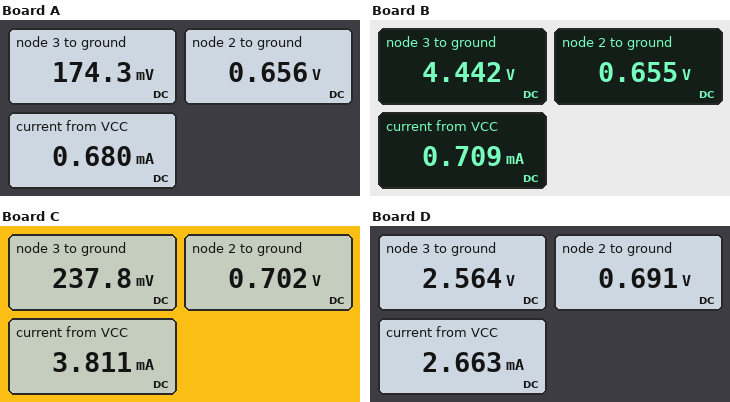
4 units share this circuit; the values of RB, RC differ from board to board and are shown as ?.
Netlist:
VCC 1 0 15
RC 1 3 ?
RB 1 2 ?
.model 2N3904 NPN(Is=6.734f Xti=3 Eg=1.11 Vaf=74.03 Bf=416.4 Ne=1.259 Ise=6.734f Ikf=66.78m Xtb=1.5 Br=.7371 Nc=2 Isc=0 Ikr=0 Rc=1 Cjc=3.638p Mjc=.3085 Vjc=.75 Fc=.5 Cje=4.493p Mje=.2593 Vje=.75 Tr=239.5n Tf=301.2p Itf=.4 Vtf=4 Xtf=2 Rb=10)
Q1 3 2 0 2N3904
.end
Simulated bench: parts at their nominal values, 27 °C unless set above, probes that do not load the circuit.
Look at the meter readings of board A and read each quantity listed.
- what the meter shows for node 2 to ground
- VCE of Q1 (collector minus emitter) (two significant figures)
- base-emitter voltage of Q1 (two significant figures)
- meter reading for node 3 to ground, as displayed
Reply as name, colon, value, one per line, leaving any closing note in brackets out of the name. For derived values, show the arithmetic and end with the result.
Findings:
what the meter shows for node 2 to ground: 0.656 V
VCE of Q1 (collector minus emitter): 174.3 mV = 170 mV
base-emitter voltage of Q1: 656 mV = 660 mV
meter reading for node 3 to ground, as displayed: 174.3 mV
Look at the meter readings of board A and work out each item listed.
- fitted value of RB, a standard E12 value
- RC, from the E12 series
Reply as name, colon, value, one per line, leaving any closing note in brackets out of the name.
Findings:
fitted value of RB, a standard E12 value: 2.2 MΩ
RC, from the E12 series: 22 kΩ
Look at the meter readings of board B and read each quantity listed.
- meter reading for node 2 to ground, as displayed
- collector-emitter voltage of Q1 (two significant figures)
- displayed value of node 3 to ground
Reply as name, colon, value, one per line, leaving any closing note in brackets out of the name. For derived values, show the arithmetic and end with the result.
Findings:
meter reading for node 2 to ground, as displayed: 0.655 V
collector-emitter voltage of Q1: 4.442 V = 4.4 V
displayed value of node 3 to ground: 4.442 V
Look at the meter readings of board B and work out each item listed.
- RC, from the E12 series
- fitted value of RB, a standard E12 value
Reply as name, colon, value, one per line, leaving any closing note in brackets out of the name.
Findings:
RC, from the E12 series: 15 kΩ
fitted value of RB, a standard E12 value: 2.7 MΩ
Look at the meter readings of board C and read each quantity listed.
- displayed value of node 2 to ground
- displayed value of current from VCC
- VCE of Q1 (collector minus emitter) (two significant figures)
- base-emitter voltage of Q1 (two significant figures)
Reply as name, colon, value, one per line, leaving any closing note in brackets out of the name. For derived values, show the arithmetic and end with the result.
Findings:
displayed value of node 2 to ground: 0.702 V
displayed value of current from VCC: 3.811 mA
VCE of Q1 (collector minus emitter): 237.8 mV = 240 mV
base-emitter voltage of Q1: 702 mV = 700 mV
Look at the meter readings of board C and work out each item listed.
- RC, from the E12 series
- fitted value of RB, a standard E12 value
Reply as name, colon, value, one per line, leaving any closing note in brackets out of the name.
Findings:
RC, from the E12 series: 3.9 kΩ
fitted value of RB, a standard E12 value: 560 kΩ
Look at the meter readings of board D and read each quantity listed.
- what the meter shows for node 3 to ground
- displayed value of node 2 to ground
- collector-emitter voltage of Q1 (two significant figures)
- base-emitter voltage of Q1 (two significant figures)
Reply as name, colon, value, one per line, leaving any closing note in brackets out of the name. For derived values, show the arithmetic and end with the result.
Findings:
what the meter shows for node 3 to ground: 2.564 V
displayed value of node 2 to ground: 0.691 V
collector-emitter voltage of Q1: 2.564 V = 2.6 V
base-emitter voltage of Q1: 691 mV = 690 mV
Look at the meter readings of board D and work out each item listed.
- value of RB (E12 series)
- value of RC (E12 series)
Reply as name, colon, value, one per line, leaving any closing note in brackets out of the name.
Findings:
value of RB: 820 kΩ
value of RC: 4.7 kΩ
